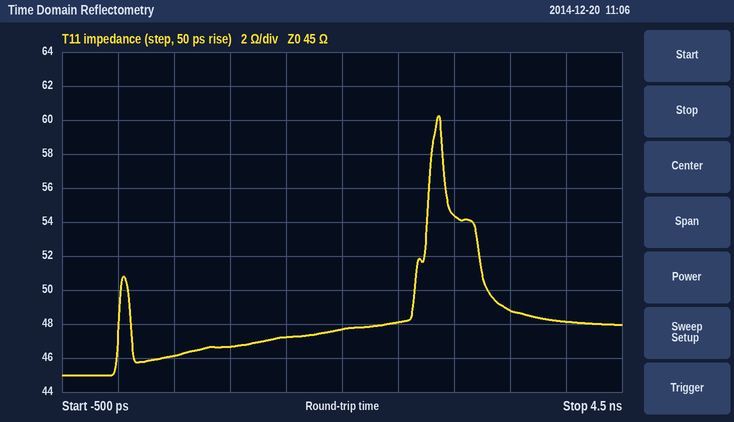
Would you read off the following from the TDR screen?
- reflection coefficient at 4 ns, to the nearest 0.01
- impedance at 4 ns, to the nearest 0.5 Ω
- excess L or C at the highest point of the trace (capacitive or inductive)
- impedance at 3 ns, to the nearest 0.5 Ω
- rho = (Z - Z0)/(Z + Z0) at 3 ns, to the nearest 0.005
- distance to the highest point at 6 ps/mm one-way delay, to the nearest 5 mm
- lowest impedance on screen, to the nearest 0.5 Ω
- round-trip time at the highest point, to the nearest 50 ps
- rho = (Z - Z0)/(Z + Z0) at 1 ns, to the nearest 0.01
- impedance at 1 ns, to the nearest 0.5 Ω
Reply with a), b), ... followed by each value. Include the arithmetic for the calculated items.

a) (48 − 45)/(48 + 45) ≈ +0.03
b) 48.0 Ω
c) inductive
d) 54.5 Ω
e) (54.5 − 45)/(54.5 + 45) ≈ +0.095
f) 2.85 ns / 2 / 6 ps/mm ≈ 238 mm, so 240 mm to the nearest 5 mm
g) 45.0 Ω
h) 2.85 ns
i) (46.5 − 45)/(46.5 + 45) ≈ +0.02
j) 46.5 Ω
